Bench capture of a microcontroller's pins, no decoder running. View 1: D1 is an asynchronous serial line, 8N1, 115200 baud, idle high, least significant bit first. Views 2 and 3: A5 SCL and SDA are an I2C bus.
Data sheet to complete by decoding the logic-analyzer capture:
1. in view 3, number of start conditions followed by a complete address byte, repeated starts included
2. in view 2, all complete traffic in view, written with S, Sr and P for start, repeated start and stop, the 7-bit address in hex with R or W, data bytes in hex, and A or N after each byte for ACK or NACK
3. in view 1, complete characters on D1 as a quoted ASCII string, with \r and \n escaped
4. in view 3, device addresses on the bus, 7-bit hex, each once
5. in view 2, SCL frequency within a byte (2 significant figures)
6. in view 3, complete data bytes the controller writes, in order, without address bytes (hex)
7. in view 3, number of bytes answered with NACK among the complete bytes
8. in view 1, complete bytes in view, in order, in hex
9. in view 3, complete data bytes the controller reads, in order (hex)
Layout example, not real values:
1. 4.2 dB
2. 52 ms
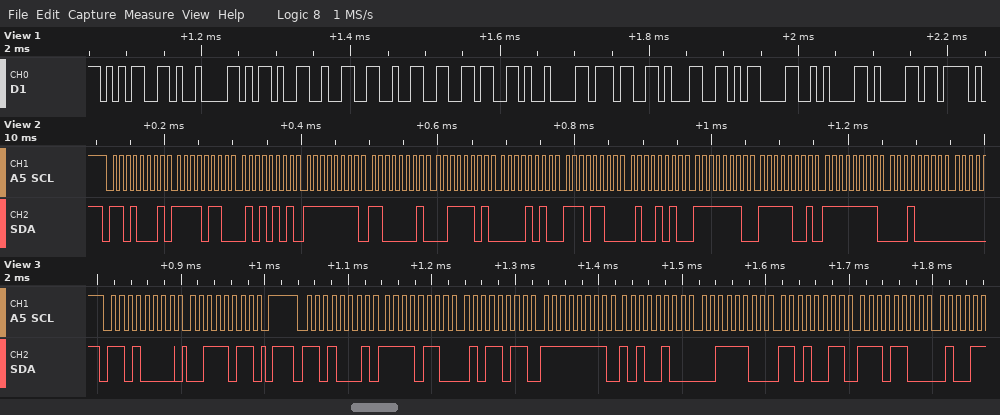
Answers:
1. 2
2. S 68R A F6 A 55 A FF A C1 A 3D A 0A A EC A 4A A FE A F9 A FF A 10 A
3. "5\t-226\t71\r\na"
4. 0x68
5. 100 kHz
6. 3B
7. 0
8. 35 09 2D 32 32 36 09 37 31 0D 0A 61
9. F6 5B FF A4 3C D3 EC
